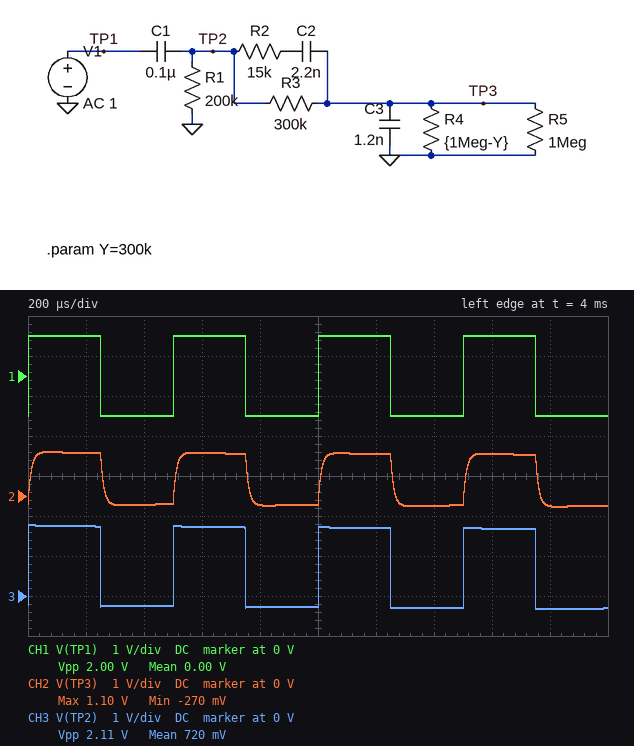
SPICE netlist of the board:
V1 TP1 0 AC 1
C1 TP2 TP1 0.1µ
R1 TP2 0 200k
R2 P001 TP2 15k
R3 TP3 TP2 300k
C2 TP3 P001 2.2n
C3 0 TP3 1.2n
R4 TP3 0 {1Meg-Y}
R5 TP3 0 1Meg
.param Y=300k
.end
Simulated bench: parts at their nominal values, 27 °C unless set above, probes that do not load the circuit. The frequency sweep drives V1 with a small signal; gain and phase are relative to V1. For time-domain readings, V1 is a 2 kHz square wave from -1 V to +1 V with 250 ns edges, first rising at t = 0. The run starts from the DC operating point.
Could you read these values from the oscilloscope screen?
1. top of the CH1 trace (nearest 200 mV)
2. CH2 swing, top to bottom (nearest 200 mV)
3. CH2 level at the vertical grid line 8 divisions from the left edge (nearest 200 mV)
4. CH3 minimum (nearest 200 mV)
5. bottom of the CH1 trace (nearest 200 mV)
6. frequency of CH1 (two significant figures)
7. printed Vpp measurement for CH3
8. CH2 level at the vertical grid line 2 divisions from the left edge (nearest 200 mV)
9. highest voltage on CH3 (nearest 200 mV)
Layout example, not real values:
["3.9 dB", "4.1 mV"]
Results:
["1.0 V", "1.4 V", "1.0 V", "-400 mV", "-1.0 V", "2.0 kHz", "2.11 V", "-200 mV", "1.8 V"]
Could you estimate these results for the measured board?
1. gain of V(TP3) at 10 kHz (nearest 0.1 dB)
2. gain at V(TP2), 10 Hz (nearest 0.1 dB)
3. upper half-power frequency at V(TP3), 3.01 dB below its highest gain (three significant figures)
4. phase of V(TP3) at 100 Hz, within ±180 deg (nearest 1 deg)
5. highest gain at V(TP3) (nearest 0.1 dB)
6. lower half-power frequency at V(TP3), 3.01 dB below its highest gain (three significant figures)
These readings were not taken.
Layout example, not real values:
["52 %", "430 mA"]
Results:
["-5.5 dB", "-3.1 dB", "14.5 kHz", "8 deg", "-3.8 dB", "13.2 Hz"]
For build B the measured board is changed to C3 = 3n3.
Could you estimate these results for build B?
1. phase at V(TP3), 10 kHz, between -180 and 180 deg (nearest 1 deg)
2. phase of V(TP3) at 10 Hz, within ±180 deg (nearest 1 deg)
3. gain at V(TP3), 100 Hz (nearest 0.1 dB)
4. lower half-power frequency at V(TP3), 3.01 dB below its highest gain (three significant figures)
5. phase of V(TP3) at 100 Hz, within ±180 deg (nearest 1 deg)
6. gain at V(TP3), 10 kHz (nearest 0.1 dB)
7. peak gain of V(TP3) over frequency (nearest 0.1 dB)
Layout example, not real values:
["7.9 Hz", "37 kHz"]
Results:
["-51 deg", "44 deg", "-5.5 dB", "9.30 Hz", "-3 deg", "-11.7 dB", "-5.2 dB"]
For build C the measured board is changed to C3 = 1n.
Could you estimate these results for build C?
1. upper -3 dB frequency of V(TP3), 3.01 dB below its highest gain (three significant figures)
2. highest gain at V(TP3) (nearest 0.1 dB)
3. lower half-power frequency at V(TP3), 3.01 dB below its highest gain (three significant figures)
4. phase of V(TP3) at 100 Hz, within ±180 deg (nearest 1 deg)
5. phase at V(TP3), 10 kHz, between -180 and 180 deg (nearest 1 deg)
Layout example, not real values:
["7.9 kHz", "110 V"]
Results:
["16.5 kHz", "-3.3 dB", "15.6 Hz", "9 deg", "-31 deg"]
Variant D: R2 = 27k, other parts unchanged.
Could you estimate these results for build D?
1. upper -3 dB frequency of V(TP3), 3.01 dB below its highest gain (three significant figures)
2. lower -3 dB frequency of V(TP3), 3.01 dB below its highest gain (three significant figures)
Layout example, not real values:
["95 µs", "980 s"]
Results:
["8.40 kHz", "13.3 Hz"]
